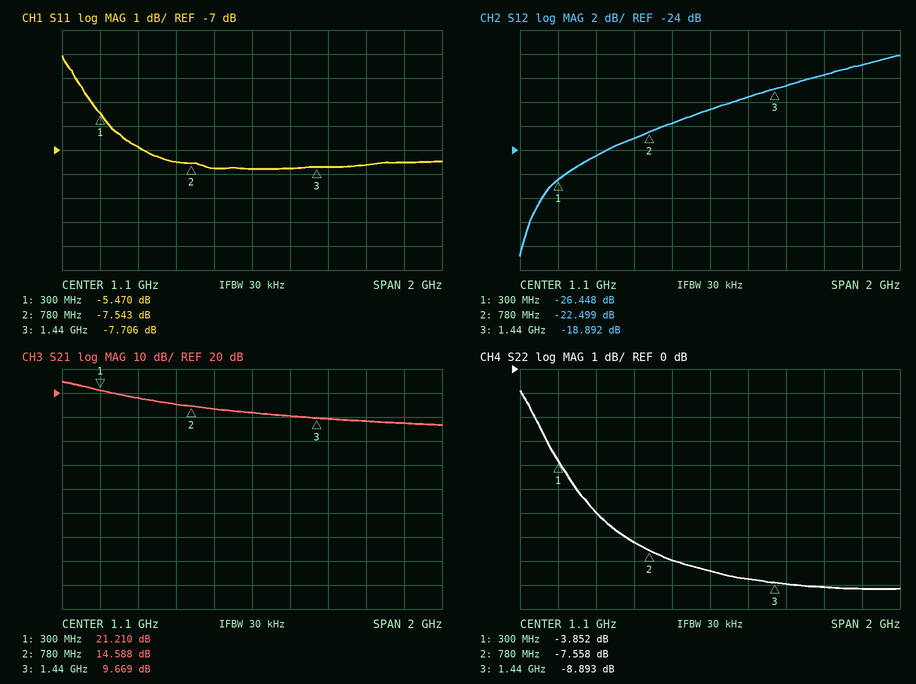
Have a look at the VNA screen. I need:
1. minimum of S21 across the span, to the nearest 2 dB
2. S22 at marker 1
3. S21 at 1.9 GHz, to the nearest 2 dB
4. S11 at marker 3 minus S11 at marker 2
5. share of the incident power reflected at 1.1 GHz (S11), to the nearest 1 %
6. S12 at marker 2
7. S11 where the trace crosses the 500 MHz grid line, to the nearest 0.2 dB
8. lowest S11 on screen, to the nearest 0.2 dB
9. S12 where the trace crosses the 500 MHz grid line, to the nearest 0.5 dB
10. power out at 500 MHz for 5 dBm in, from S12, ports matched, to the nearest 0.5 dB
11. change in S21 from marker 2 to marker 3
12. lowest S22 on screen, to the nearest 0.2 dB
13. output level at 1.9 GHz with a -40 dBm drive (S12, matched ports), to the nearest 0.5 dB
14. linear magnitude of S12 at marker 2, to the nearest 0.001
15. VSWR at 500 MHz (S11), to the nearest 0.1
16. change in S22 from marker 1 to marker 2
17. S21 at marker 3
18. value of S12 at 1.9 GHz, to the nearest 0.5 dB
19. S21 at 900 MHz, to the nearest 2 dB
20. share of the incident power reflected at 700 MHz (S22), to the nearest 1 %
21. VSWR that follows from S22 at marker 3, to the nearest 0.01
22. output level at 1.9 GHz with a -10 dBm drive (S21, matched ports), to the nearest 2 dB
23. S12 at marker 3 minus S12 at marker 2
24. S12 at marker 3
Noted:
6 dB
-3.852 dB
8 dB
-0.163 dB
17 %
-22.499 dB
-6.8 dB
-7.8 dB
-24.5 dB
-19.5 dBm
-4.919 dB
-9.2 dB
-57.0 dBm
0.075
2.7
-3.706 dB
9.669 dB
-17.0 dB
14 dB
19 %
2.12
-2 dBm
3.607 dB
-18.892 dB
